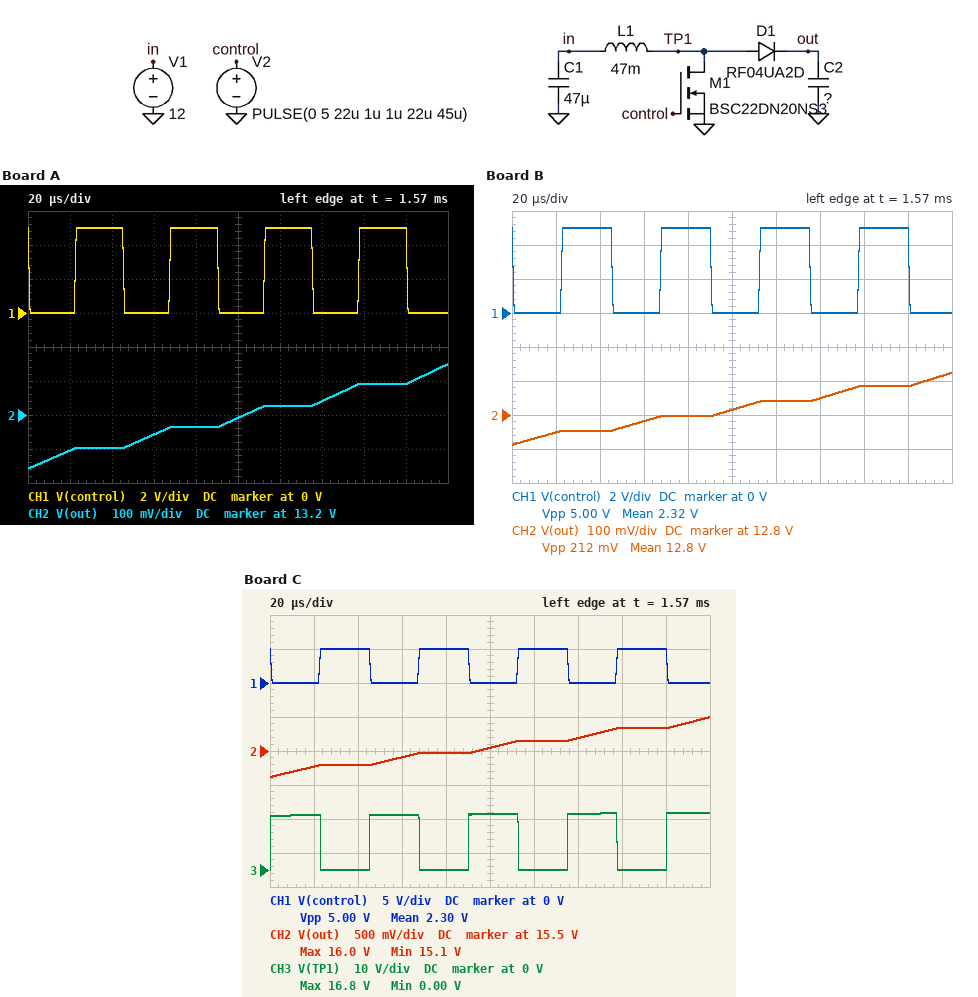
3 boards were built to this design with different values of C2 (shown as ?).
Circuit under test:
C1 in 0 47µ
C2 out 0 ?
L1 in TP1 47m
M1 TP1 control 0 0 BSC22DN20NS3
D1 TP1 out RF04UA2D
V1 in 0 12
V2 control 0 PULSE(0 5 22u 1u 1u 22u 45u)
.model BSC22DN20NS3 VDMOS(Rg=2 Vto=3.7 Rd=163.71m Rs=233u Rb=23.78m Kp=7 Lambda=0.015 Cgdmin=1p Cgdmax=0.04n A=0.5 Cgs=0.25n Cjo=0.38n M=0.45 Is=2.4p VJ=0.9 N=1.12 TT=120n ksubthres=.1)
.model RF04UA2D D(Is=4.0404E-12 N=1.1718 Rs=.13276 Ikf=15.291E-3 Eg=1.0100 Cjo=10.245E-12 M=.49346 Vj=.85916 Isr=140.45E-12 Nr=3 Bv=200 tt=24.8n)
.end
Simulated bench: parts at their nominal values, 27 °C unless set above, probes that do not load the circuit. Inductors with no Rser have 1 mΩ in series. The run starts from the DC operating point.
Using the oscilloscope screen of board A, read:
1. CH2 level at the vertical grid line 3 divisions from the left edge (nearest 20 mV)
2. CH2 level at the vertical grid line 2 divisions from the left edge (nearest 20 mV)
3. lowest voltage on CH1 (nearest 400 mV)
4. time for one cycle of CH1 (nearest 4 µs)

13.14 V
13.10 V
0 V
44 µs
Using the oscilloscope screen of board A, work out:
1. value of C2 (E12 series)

68 µF
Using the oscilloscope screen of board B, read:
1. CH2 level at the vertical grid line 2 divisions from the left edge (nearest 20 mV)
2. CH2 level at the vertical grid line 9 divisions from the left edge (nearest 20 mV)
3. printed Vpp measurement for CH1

12.76 V
12.88 V
5.00 V
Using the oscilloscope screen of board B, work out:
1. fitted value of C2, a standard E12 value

100 µF
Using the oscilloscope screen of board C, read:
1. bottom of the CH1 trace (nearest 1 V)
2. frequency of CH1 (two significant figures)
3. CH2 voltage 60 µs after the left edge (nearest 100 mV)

0 V
22 kHz
15.4 V
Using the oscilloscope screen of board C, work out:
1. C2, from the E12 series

22 µF
